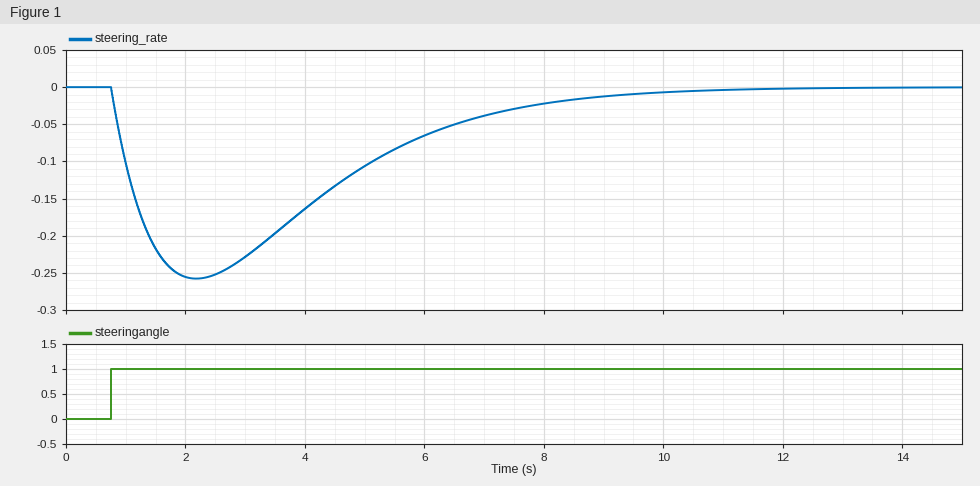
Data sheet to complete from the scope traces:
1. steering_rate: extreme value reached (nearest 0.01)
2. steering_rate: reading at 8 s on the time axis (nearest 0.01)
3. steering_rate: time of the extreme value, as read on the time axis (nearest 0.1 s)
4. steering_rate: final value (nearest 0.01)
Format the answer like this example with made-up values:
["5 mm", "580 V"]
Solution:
["-0.26", "-0.02", "2.2 s", "0.00"]
